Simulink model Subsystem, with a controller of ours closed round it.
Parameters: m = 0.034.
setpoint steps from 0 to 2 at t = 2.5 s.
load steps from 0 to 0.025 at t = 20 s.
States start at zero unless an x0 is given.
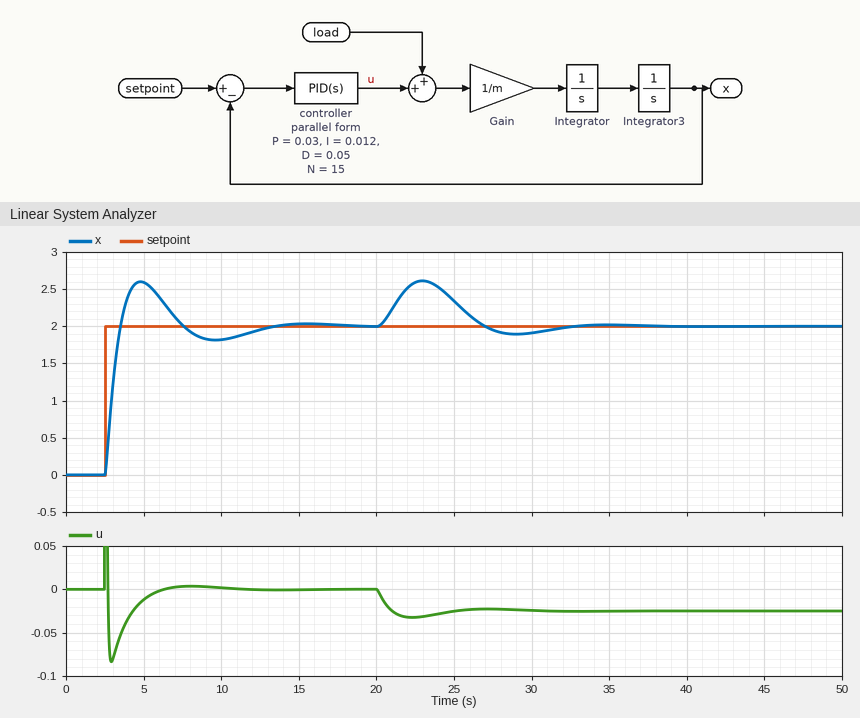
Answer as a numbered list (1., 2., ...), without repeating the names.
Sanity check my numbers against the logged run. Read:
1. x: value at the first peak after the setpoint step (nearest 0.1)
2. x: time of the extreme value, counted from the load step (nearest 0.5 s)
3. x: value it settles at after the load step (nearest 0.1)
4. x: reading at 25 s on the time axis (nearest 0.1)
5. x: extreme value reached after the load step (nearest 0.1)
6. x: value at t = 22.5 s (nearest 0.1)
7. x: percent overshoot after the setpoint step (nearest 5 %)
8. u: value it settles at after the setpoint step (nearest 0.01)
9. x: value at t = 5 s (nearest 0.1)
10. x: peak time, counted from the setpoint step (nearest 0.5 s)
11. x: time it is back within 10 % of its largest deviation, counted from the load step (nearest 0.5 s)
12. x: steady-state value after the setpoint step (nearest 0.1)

1. 2.6
2. 3.0 s
3. 2.0
4. 2.3
5. 2.6
6. 2.6
7. 30 %
8. 0.00
9. 2.6
10. 2.5 s
11. 11.0 s
12. 2.0
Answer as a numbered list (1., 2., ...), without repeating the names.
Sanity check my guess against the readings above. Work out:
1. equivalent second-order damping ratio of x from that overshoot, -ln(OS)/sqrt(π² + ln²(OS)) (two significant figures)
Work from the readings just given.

1. 0.36
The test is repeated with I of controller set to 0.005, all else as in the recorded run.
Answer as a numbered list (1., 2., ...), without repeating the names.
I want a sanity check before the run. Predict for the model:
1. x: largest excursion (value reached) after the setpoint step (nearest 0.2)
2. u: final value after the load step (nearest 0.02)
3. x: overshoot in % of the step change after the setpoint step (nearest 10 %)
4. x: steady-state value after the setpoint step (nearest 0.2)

1. 2.4
2. -0.02
3. 20 %
4. 2.0
